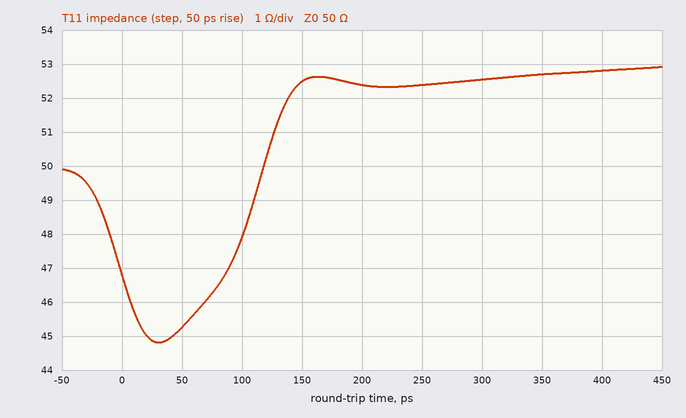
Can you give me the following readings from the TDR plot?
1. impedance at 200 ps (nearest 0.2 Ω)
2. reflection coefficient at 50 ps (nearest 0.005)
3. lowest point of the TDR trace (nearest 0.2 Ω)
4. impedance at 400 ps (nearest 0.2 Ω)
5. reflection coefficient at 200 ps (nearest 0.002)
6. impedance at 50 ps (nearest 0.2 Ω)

52.4 Ω
-0.050
44.8 Ω
52.8 Ω
+0.024
45.2 Ω
